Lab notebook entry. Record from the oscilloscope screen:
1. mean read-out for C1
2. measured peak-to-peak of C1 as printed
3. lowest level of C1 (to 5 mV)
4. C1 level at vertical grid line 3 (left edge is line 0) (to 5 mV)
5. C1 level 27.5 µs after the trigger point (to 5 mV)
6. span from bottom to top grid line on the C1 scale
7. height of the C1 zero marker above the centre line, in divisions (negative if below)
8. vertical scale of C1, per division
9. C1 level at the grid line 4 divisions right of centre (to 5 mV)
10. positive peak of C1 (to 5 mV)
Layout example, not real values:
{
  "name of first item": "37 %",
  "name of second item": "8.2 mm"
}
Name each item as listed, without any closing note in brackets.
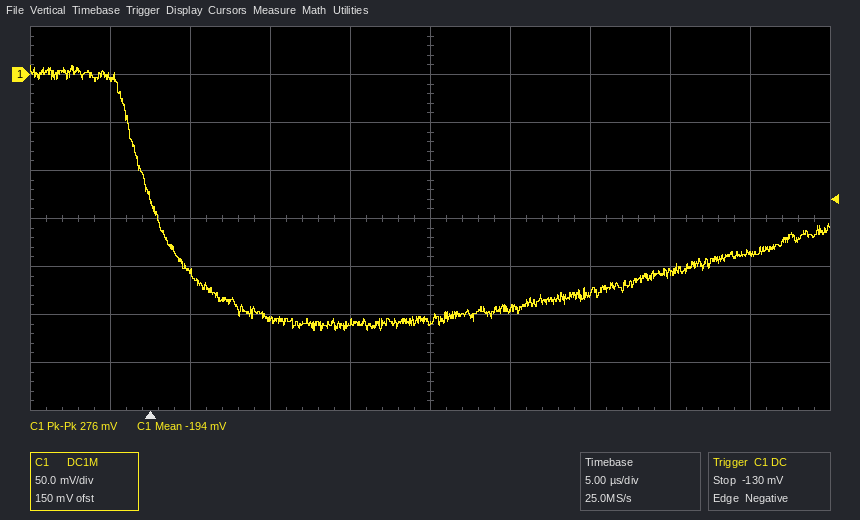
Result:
{
  "mean read-out for C1": "-194 mV",
  "measured peak-to-peak of C1 as printed": "276 mV",
  "lowest level of C1": "-265 mV",
  "C1 level at vertical grid line 3 (left edge is line 0)": "-255 mV",
  "C1 level 27.5 µs after the trigger point": "-225 mV",
  "span from bottom to top grid line on the C1 scale": "400 mV",
  "height of the C1 zero marker above the centre line, in divisions": "+3.0 div",
  "vertical scale of C1, per division": "50 mV",
  "C1 level at the grid line 4 divisions right of centre": "-185 mV",
  "positive peak of C1": "10 mV"
}
